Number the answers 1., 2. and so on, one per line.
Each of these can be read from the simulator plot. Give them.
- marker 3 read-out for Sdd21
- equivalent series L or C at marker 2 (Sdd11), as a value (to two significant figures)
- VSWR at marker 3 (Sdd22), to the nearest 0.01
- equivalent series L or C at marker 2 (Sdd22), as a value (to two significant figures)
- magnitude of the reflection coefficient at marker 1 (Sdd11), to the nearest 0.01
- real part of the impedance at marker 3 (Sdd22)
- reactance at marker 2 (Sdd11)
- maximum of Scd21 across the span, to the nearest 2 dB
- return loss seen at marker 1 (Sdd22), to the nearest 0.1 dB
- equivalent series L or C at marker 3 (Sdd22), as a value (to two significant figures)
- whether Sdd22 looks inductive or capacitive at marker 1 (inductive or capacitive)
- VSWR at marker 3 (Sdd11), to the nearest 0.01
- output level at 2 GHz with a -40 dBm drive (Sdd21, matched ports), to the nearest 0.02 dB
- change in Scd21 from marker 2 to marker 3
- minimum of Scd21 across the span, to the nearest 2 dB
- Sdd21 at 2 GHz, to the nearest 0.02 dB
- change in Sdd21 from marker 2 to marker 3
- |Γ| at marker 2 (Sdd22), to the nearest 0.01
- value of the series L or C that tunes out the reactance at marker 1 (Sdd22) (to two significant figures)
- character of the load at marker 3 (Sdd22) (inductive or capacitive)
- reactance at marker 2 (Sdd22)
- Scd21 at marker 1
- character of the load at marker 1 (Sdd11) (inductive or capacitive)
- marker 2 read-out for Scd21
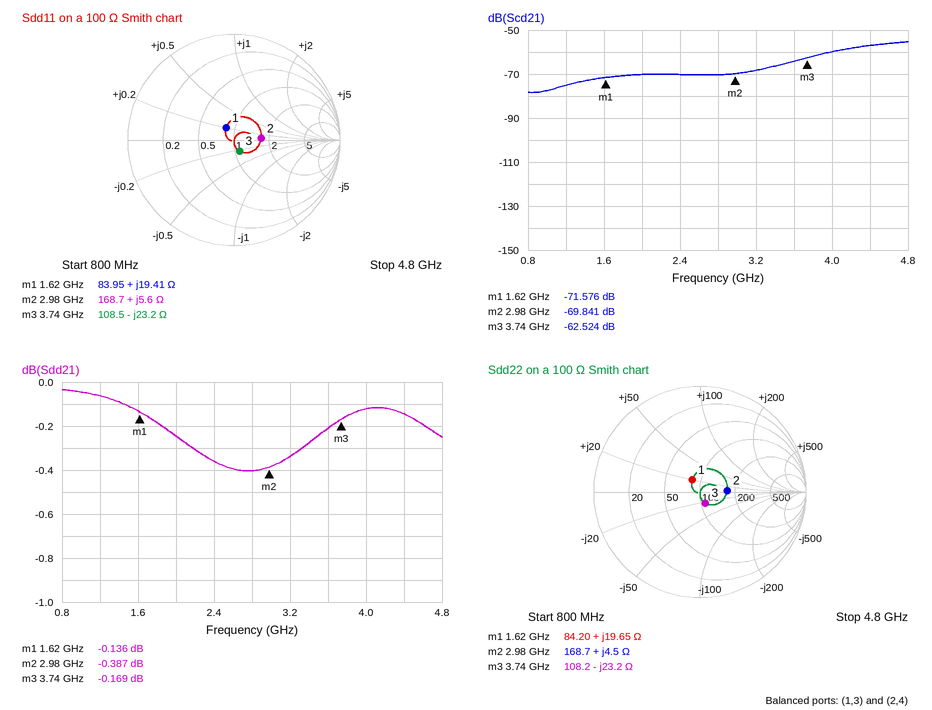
1. -0.169 dB
2. 300 pH
3. 1.27
4. 240 pH
5. 0.14
6. 108.2 Ω
7. +5.6 Ω
8. -56 dB
9. 17.3 dB
10. 1.8 pF
11. inductive
12. 1.27
13. -40.24 dBm
14. 7.317 dB
15. -78 dB
16. -0.24 dB
17. 0.218 dB
18. 0.26
19. 5.0 pF
20. capacitive
21. +4.5 Ω
22. -71.576 dB
23. inductive
24. -69.841 dB
